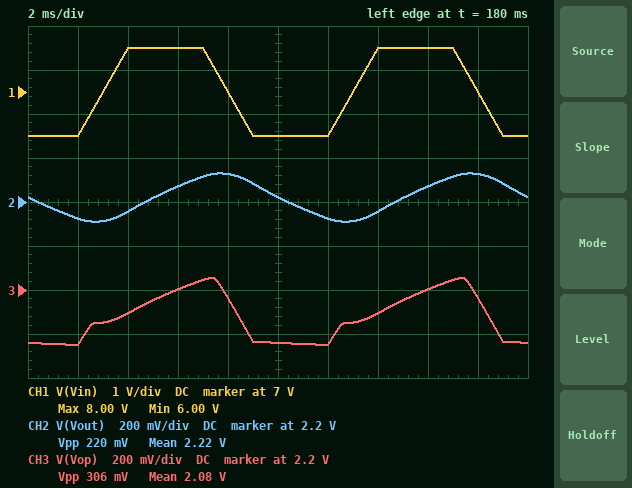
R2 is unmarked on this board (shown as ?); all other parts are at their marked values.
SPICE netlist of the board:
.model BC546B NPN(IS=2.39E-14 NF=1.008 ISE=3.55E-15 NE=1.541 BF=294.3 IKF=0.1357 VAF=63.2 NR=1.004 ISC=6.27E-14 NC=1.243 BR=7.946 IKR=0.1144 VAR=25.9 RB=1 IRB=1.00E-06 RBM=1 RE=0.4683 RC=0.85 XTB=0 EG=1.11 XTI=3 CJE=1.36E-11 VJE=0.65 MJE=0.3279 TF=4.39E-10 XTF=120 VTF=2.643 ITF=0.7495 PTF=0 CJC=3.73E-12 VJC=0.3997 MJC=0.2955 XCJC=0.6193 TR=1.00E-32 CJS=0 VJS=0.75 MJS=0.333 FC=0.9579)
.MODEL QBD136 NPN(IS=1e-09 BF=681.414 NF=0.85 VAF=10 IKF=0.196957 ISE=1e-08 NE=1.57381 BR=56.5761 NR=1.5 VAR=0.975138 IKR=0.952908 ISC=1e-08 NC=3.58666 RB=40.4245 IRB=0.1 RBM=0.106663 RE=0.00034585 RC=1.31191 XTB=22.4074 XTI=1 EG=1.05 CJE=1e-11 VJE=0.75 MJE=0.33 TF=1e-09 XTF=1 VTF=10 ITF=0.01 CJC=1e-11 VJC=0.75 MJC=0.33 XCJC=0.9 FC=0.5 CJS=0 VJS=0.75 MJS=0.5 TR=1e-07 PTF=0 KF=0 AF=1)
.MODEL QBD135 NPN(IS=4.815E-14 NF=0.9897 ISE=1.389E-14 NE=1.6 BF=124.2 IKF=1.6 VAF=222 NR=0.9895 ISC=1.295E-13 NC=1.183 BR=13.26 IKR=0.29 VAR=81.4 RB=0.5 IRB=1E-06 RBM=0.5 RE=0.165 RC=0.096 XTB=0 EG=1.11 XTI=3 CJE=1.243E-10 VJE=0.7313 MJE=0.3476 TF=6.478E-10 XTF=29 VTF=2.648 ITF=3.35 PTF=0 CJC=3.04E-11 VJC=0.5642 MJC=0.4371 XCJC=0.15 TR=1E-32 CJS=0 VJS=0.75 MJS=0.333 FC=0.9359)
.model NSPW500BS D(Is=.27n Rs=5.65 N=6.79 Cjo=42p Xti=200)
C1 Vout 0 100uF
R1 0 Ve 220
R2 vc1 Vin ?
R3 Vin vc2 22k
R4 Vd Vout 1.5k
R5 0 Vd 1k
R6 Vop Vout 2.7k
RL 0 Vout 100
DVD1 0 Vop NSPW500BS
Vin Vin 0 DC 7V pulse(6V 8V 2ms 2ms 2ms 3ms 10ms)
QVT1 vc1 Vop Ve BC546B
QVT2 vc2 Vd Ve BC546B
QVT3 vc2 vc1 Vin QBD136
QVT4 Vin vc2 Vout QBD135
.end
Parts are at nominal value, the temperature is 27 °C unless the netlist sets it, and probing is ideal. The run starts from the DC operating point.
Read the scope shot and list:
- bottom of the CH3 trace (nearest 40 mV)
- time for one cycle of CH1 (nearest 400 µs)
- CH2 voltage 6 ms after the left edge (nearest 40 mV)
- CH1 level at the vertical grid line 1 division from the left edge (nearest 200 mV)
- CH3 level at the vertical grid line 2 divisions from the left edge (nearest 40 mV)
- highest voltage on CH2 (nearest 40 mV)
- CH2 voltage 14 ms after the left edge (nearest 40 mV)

1.96 V
10.0 ms
2.28 V
6.0 V
2.08 V
2.32 V
2.16 V
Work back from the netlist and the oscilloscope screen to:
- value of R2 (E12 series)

820 Ω
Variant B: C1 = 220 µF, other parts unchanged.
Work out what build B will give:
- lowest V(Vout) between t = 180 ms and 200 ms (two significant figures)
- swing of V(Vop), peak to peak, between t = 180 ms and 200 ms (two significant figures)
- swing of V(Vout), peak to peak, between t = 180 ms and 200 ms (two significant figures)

2.2 V
250 mV
100 mV
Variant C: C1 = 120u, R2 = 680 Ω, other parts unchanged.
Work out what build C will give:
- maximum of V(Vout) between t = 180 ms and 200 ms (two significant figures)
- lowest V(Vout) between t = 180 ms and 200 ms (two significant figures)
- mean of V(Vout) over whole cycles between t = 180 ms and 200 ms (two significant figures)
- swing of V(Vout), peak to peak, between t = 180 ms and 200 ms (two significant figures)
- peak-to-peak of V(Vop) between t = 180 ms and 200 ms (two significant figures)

2.4 V
2.2 V
2.3 V
220 mV
210 mV
